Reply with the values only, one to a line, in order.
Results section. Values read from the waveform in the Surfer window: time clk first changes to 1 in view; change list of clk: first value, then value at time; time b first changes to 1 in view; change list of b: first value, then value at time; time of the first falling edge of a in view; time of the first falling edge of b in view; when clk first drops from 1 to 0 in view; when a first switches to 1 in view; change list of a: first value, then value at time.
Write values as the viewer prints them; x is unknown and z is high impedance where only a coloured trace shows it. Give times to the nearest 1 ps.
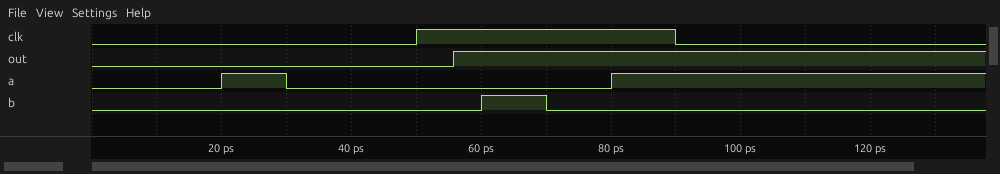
50 ps
0, 1 at 50 ps, 0 at 90 ps
60 ps
0, 1 at 60 ps, 0 at 70 ps
30 ps
70 ps
90 ps
20 ps
0, 1 at 20 ps, 0 at 30 ps, 1 at 80 ps
